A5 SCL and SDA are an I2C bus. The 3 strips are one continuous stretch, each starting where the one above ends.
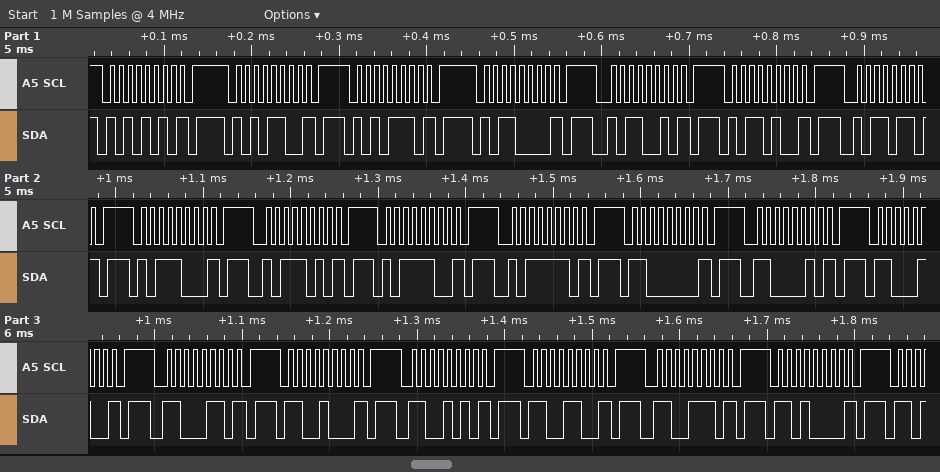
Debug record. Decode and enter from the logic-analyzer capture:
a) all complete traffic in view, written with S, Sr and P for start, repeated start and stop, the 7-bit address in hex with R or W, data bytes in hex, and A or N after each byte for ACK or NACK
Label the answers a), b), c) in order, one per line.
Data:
a) S 55W N P S 56W N P S 57W N P S 58W N P S 59W N P S 5AW N P S 5BW N P S 5CW N P S 5DW N P S 5EW N P S 5FW N P S 60W N P S 61W N P S 62W N P S 63W N P S 64W N P S 65W N P S 66W N P S 67W N P S 68W N P
